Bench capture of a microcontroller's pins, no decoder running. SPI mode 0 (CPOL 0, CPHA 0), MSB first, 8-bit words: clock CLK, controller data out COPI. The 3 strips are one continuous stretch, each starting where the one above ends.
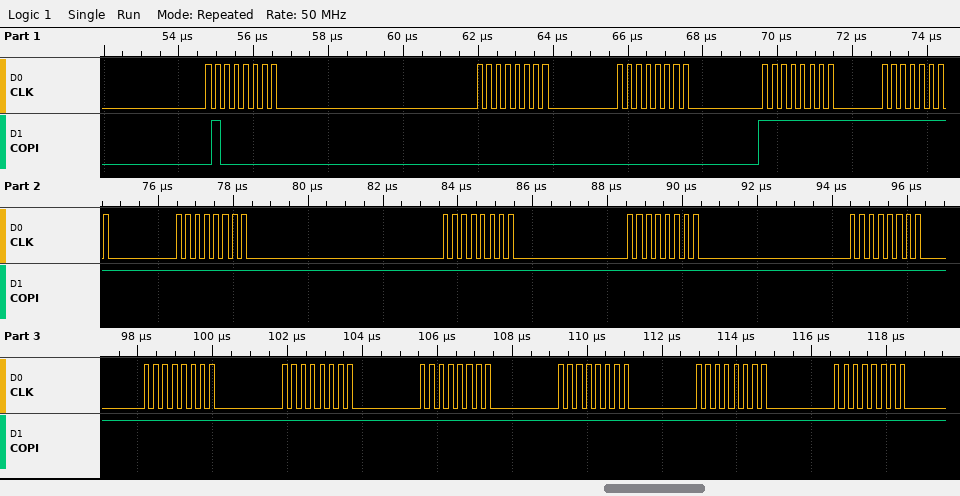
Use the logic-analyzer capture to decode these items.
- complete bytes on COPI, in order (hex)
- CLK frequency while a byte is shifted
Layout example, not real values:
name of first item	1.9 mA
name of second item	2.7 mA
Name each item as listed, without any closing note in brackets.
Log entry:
complete bytes on COPI, in order	0x40 0x00 0x00 0xFF 0xFF 0xFF 0xFF 0xFF 0xFF 0xFF 0xFF 0xFF 0xFF 0xFF 0xFF
CLK frequency while a byte is shifted	4 MHz
